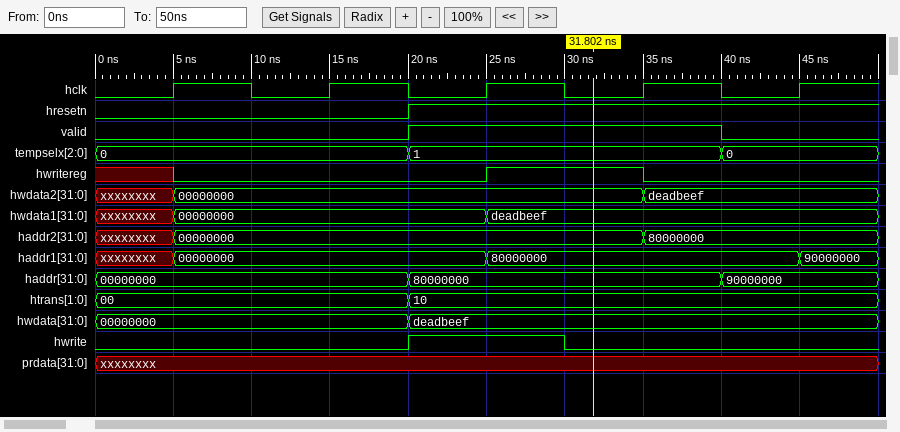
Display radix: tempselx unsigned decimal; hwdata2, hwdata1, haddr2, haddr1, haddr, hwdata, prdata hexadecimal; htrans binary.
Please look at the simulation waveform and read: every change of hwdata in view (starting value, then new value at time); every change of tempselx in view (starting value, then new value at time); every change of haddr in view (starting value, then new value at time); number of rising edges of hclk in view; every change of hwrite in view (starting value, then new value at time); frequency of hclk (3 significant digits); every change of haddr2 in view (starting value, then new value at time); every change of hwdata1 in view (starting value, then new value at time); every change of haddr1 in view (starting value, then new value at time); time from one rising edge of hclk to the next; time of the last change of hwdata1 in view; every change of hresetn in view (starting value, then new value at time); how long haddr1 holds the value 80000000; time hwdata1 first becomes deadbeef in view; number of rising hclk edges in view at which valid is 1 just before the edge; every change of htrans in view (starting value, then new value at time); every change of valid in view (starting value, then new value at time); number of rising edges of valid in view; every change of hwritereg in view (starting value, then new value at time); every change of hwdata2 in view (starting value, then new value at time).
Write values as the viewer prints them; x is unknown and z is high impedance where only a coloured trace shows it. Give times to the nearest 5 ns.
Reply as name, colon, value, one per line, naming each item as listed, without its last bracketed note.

every change of hwdata in view: 00000000, deadbeef at 20 ns
every change of tempselx in view: 0, 1 at 20 ns, 0 at 40 ns
every change of haddr in view: 00000000, 80000000 at 20 ns, 90000000 at 40 ns
number of rising edges of hclk in view: 5
every change of hwrite in view: 0, 1 at 20 ns, 0 at 30 ns
frequency of hclk: 100 MHz
every change of haddr2 in view: xxxxxxxx, 00000000 at 5 ns, 80000000 at 35 ns
every change of hwdata1 in view: xxxxxxxx, 00000000 at 5 ns, deadbeef at 25 ns
every change of haddr1 in view: xxxxxxxx, 00000000 at 5 ns, 80000000 at 25 ns, 90000000 at 45 ns
time from one rising edge of hclk to the next: 10 ns
time of the last change of hwdata1 in view: 25 ns
every change of hresetn in view: 0, 1 at 20 ns
how long haddr1 holds the value 80000000: 20 ns
time hwdata1 first becomes deadbeef in view: 25 ns
number of rising hclk edges in view at which valid is 1 just before the edge: 2
every change of htrans in view: 00, 10 at 20 ns
every change of valid in view: 0, 1 at 20 ns, 0 at 40 ns
number of rising edges of valid in view: 1
every change of hwritereg in view: x, 0 at 5 ns, 1 at 25 ns, 0 at 35 ns
every change of hwdata2 in view: xxxxxxxx, 00000000 at 5 ns, deadbeef at 35 ns
